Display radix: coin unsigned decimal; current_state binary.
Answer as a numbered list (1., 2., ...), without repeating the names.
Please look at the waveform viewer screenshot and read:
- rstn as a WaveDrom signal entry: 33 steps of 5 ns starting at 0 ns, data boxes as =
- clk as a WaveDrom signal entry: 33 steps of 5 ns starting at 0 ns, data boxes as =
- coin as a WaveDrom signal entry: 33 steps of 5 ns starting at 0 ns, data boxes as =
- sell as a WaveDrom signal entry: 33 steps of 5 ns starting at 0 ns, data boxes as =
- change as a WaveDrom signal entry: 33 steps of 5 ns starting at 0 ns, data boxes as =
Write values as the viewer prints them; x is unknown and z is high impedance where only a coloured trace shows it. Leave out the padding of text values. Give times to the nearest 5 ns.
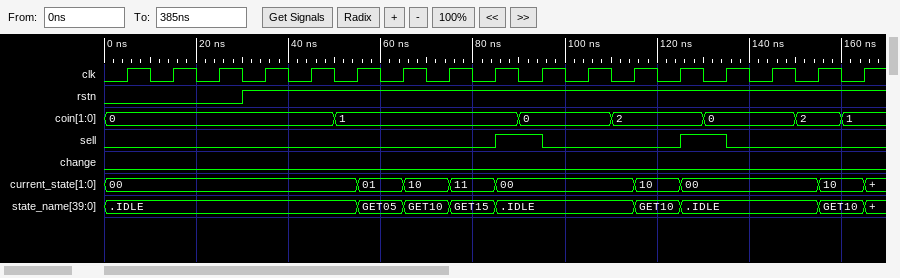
1. {name: 'rstn', wave: '0.....1..........................'}
2. {name: 'clk', wave: '010101010101010101010101010101010'}
3. {name: 'coin', wave: '=.........=.......=...=...=...=.=', data: '0 1 0 2 0 2 1'}
4. {name: 'sell', wave: '0................1.0.....1.0.....'}
5. {name: 'change', wave: '0................................'}
